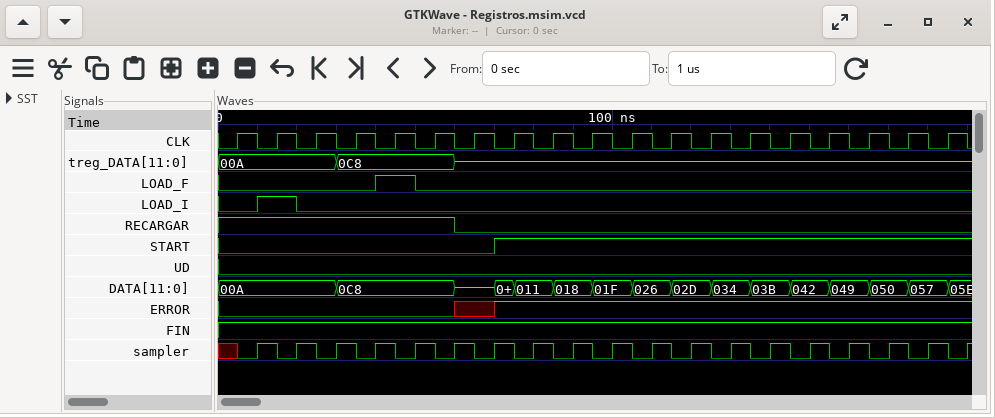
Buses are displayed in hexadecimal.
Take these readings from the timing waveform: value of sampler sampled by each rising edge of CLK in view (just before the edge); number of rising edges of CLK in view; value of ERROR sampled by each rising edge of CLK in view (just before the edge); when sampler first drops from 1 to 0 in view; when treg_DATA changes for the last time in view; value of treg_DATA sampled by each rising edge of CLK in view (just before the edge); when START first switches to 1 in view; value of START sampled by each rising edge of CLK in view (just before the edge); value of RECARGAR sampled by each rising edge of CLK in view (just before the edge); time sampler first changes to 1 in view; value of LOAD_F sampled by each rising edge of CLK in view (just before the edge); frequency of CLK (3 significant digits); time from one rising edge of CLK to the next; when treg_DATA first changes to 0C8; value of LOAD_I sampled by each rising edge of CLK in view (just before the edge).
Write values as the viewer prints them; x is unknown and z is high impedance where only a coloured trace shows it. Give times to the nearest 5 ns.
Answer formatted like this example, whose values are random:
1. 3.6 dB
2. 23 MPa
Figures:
1. x 1 1 1 1 1 1 1 1 1 1 1 1 1 1 1 1 1 1
2. 19
3. 0 0 0 0 0 0 x 1 1 1 1 1 1 1 1 1 1 1 1
4. 15 ns
5. 60 ns
6. 00A, 00A, 00A, 0C8, 0C8, 0C8, z, z, z, z, z, z, z, z, z, z, z, z, z
7. 70 ns
8. 0 0 0 0 0 0 0 1 1 1 1 1 1 1 1 1 1 1 1
9. 1 1 1 1 1 1 0 0 0 0 0 0 0 0 0 0 0 0 0
10. 10 ns
11. 0 0 0 0 1 0 0 0 0 0 0 0 0 0 0 0 0 0 0
12. 100 MHz
13. 10 ns
14. 30 ns
15. 0 1 0 0 0 0 0 0 0 0 0 0 0 0 0 0 0 0 0
